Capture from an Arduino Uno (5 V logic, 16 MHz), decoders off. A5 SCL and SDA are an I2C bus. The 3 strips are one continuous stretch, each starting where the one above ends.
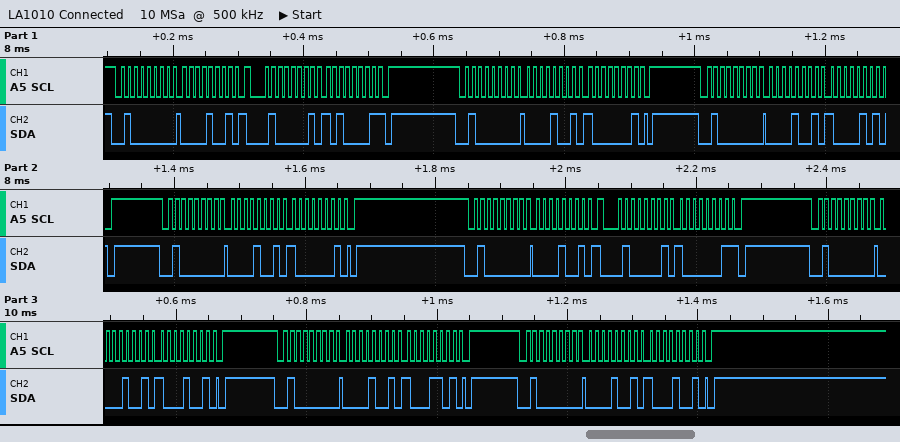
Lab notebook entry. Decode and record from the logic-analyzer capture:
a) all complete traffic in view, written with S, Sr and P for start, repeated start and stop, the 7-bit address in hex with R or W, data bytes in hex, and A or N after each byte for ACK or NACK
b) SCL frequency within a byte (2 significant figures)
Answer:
S 20W A 09 A Sr 20R A A1 N P S 20W A 09 A 81 A P S 20W A 09 A 85 A P S 20W A 09 A 81 A P S 20W A 09 A Sr 20R A 81 N P S 20W A 09 A 89 A P S 20W A 09 A 8D A P S 20W A 09 A 89 A P
100 kHz
